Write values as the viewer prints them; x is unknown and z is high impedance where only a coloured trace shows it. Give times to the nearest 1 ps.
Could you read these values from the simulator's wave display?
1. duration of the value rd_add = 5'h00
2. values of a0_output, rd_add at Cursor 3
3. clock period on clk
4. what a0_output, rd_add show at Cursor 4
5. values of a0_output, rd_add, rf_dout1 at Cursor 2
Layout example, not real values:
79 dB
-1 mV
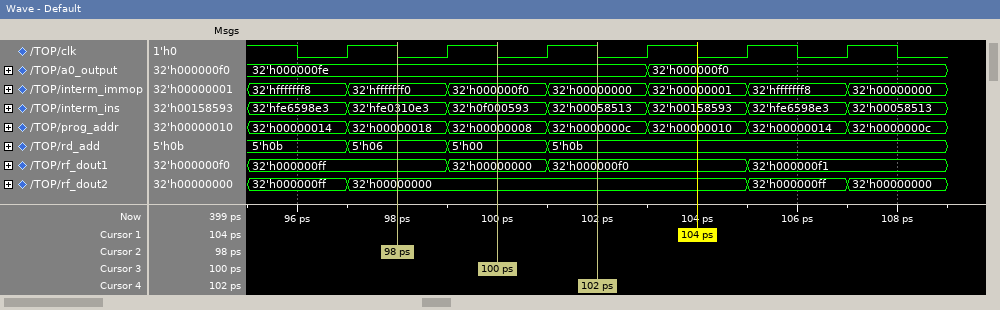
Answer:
2 ps
a0_output=32'h000000fe, rd_add=5'h00
2 ps
a0_output=32'h000000fe, rd_add=5'h0b
a0_output=32'h000000fe, rd_add=5'h06, rf_dout1=32'h000000ff
